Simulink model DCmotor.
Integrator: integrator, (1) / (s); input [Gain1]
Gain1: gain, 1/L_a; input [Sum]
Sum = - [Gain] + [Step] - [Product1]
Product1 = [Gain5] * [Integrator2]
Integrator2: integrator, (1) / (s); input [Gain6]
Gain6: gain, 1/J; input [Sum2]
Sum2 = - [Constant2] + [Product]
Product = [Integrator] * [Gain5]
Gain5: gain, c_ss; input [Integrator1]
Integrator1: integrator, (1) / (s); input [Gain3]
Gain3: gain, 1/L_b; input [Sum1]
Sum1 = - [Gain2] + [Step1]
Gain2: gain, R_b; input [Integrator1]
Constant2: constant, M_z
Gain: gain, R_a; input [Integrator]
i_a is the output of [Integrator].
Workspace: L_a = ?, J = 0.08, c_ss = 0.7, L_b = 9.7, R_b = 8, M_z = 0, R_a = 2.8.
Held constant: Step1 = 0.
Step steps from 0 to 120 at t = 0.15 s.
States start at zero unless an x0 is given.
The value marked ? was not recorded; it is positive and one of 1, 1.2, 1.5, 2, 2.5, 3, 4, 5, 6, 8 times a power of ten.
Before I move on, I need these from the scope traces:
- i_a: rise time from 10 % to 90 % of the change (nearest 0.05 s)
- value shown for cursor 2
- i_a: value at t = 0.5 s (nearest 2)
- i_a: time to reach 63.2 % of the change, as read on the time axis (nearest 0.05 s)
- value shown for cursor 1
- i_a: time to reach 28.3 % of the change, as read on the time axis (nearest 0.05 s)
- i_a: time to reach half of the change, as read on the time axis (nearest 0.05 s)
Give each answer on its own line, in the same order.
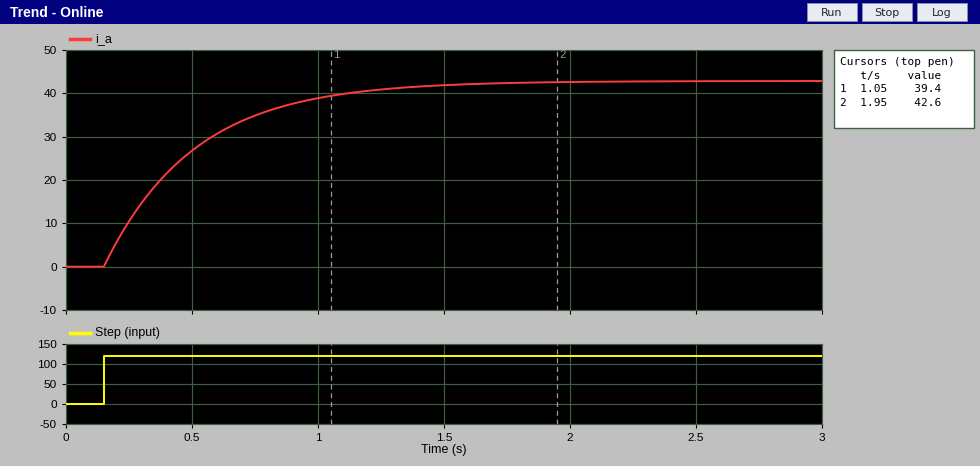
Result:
0.80 s
42.6
26
0.50 s
39.4
0.25 s
0.40 s
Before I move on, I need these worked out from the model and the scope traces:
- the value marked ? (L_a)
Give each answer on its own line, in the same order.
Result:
1
